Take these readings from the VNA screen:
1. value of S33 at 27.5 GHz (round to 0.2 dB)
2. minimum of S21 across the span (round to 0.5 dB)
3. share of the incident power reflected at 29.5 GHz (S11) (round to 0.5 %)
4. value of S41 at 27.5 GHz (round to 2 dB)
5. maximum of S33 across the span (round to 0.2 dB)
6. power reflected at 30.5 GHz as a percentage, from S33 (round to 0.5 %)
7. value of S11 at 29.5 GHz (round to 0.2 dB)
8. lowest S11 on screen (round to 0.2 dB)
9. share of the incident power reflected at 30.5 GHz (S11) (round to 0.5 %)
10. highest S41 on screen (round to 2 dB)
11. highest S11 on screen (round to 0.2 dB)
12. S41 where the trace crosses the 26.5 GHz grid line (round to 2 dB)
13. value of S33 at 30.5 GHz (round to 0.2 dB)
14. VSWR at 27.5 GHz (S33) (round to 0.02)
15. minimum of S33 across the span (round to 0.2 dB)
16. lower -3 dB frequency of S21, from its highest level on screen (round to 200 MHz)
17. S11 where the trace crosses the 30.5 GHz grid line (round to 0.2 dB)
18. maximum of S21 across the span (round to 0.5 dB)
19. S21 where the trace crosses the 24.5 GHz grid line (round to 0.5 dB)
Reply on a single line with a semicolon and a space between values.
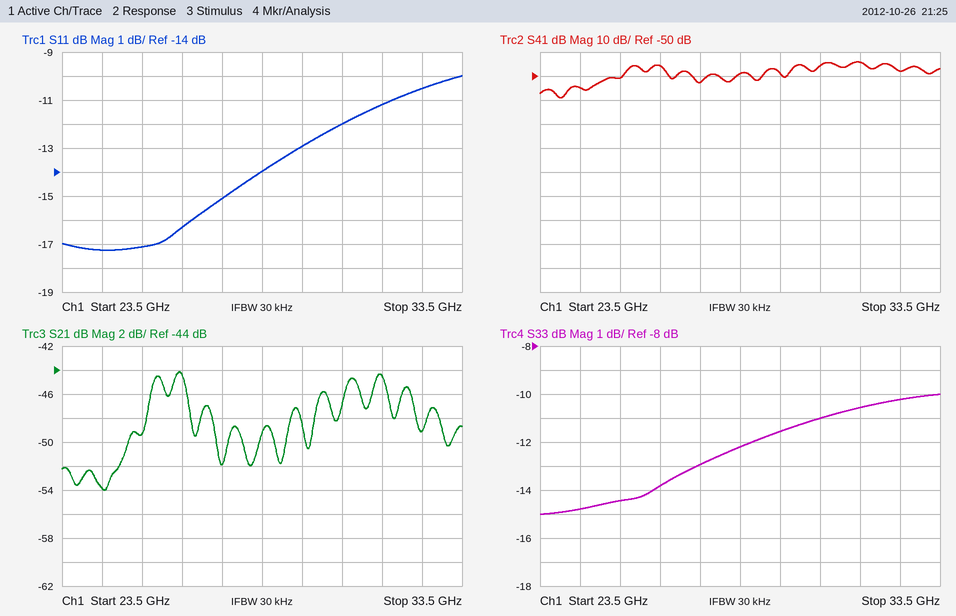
-13.0 dB; -54.0 dB; 5.0 %; -52 dB; -10.0 dB; 8.0 %; -13.0 dB; -17.2 dB; 6.5 %; -44 dB; -10.0 dB; -46 dB; -11.0 dB; 1.58; -15.0 dB; 25.6 GHz; -12.0 dB; -44.0 dB; -54.0 dB
